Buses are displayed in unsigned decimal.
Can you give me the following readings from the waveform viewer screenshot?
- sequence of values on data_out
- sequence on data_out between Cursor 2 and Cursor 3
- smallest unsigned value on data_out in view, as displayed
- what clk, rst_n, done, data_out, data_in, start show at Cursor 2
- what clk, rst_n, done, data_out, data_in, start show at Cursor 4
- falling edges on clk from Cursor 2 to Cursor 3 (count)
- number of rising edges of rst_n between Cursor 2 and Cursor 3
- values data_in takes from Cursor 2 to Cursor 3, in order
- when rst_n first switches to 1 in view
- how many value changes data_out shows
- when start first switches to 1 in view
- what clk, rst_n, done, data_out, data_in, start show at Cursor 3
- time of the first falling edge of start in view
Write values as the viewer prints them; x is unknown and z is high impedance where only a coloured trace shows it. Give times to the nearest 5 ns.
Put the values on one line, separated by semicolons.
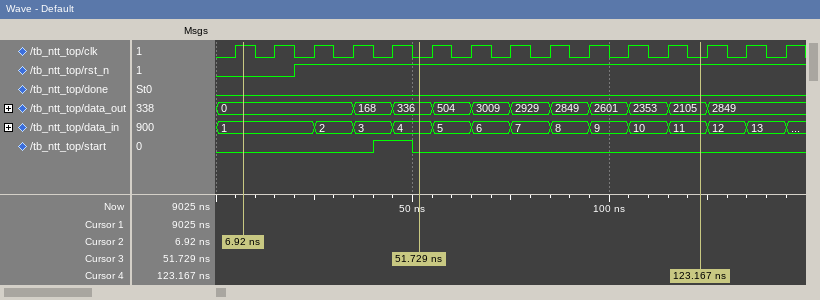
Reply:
0, 168, 336, 504, 3009, 2929, 2849, 2601, 2353, 2105, 2849; 0, 168, 336; 0; clk=1, rst_n=0, done=0, data_out=0, data_in=1, start=0; clk=0, rst_n=1, done=0, data_out=2105, data_in=11, start=0; 5; 1; 1, 2, 3, 4; 20 ns; 10; 40 ns; clk=0, rst_n=1, done=0, data_out=336, data_in=4, start=0; 50 ns
